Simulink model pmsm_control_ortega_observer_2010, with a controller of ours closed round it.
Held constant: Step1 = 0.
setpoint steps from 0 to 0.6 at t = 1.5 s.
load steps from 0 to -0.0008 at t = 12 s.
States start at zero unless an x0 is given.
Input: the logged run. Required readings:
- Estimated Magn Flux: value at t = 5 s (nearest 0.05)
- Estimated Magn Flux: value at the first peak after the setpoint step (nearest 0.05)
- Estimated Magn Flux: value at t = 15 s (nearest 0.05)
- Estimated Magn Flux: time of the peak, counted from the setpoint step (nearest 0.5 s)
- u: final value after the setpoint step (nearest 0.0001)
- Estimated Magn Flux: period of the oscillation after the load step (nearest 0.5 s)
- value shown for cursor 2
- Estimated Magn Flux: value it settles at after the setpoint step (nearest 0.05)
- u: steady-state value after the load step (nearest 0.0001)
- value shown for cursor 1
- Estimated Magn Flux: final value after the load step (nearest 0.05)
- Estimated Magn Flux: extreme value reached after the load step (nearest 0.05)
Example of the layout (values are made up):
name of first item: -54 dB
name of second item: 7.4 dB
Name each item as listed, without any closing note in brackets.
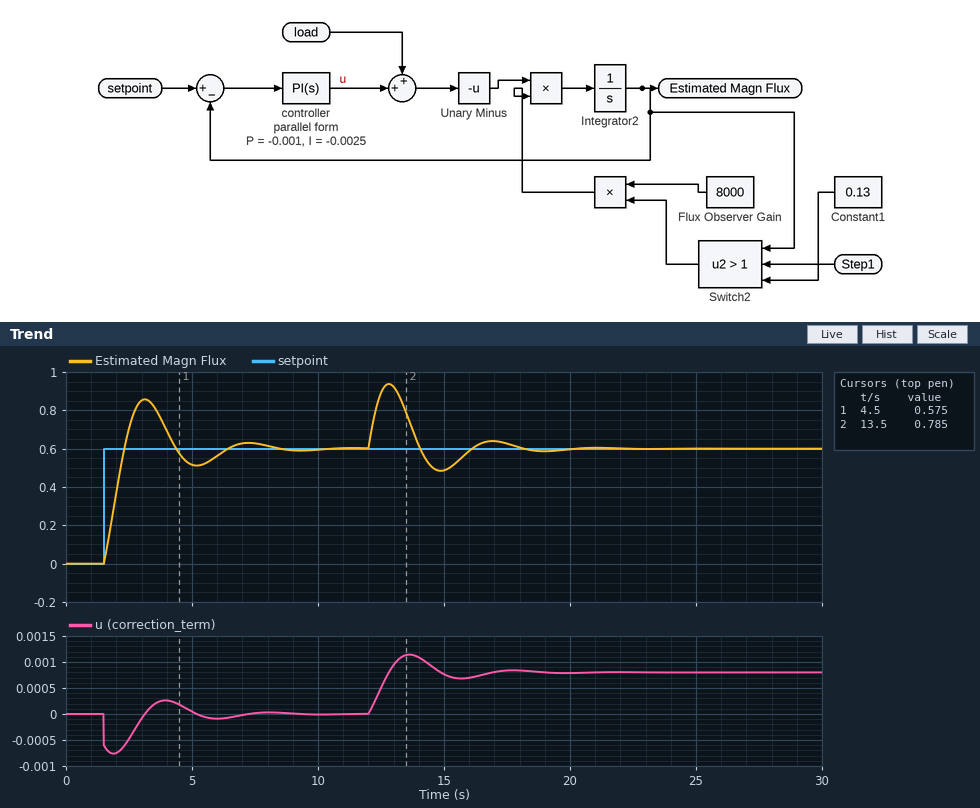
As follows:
Estimated Magn Flux: value at t = 5 s: 0.50
Estimated Magn Flux: value at the first peak after the setpoint step: 0.85
Estimated Magn Flux: value at t = 15 s: 0.50
Estimated Magn Flux: time of the peak, counted from the setpoint step: 1.5 s
u: final value after the setpoint step: 0.0000
Estimated Magn Flux: period of the oscillation after the load step: 4.0 s
value shown for cursor 2: 0.785
Estimated Magn Flux: value it settles at after the setpoint step: 0.60
u: steady-state value after the load step: 0.0008
value shown for cursor 1: 0.575
Estimated Magn Flux: final value after the load step: 0.60
Estimated Magn Flux: extreme value reached after the load step: 0.95
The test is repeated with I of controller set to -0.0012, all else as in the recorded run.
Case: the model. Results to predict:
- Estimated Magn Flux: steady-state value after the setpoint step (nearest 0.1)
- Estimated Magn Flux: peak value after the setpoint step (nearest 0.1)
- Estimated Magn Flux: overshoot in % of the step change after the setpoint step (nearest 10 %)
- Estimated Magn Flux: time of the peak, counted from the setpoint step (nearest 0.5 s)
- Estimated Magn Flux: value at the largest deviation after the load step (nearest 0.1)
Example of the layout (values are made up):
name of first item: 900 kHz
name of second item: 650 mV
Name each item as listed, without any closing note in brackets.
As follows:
Estimated Magn Flux: steady-state value after the setpoint step: 0.6
Estimated Magn Flux: peak value after the setpoint step: 0.8
Estimated Magn Flux: overshoot in % of the step change after the setpoint step: 30 %
Estimated Magn Flux: time of the peak, counted from the setpoint step: 2.0 s
Estimated Magn Flux: value at the largest deviation after the load step: 1.0
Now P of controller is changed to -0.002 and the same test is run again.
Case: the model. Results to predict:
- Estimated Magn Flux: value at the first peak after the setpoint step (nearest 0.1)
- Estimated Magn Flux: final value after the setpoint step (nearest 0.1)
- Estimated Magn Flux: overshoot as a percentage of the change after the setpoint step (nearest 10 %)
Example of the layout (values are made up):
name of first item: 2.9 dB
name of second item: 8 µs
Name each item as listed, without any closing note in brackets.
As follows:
Estimated Magn Flux: value at the first peak after the setpoint step: 0.7
Estimated Magn Flux: final value after the setpoint step: 0.6
Estimated Magn Flux: overshoot as a percentage of the change after the setpoint step: 20 %
